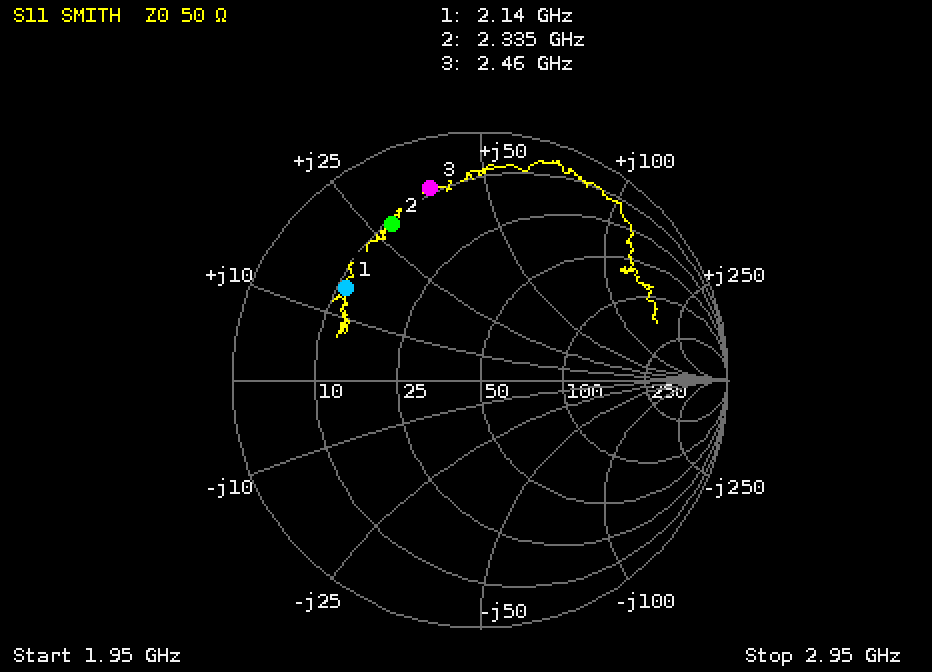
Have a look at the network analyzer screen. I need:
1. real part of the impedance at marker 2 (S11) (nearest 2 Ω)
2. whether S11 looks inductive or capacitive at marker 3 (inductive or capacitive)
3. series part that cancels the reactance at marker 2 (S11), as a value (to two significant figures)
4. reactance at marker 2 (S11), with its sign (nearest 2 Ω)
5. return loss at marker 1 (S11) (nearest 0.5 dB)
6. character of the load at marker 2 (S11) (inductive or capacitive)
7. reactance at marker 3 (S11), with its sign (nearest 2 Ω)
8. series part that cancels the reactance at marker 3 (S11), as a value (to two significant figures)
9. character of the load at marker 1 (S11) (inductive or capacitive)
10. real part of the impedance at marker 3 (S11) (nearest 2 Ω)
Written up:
10 Ω
inductive
2.4 pF
+28 Ω
3.5 dB
inductive
+38 Ω
1.7 pF
inductive
8 Ω
